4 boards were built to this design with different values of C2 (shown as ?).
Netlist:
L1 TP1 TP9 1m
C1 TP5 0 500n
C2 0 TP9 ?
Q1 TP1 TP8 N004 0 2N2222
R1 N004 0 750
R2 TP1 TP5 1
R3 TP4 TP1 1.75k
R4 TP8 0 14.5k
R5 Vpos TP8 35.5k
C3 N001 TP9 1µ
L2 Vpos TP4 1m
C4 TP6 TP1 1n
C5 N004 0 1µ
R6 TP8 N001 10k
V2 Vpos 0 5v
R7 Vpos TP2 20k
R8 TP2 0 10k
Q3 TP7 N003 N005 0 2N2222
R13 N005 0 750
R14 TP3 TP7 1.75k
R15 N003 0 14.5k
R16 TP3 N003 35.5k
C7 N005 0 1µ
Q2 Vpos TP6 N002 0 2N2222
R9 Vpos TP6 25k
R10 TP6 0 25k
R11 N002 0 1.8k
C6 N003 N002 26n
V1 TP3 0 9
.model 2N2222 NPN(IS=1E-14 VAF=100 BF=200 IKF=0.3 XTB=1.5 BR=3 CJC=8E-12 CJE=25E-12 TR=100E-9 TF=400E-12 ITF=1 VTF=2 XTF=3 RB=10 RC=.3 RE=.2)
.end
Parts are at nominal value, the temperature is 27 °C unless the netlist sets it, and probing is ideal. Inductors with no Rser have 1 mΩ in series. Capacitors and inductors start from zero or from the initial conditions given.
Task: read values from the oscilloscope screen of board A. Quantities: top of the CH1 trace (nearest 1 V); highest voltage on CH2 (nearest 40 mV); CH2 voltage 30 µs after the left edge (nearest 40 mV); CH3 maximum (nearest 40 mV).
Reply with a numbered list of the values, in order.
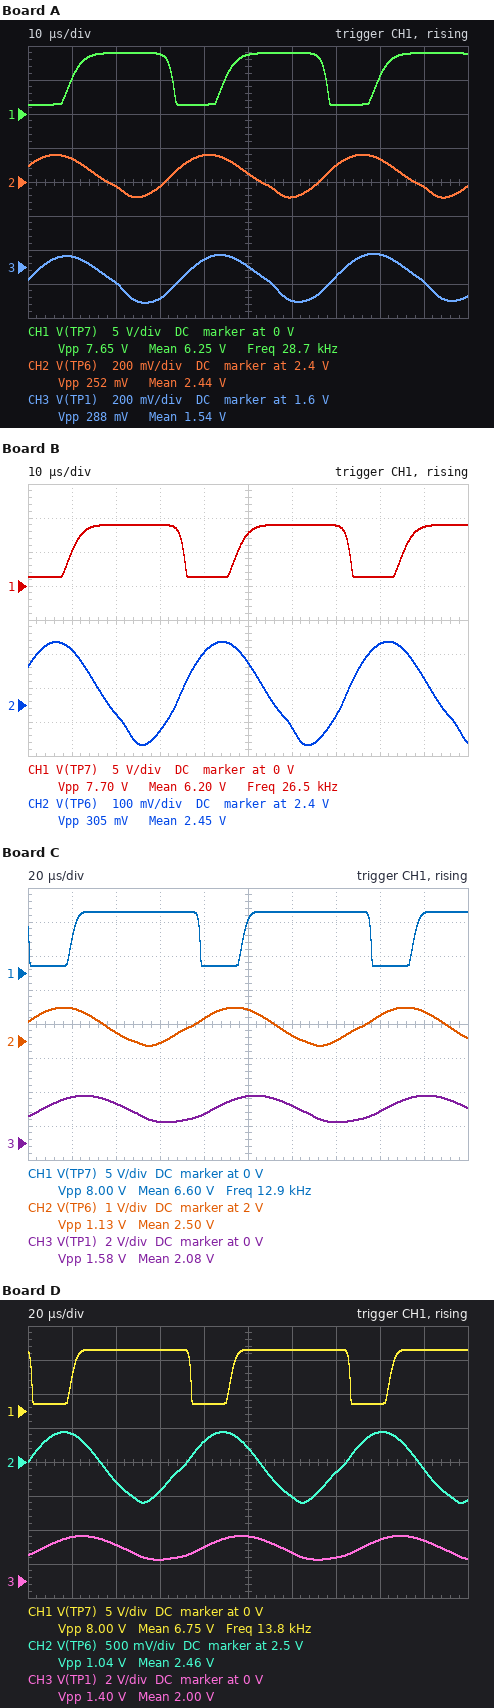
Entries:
1. 9 V
2. 2.56 V
3. 2.36 V
4. 1.68 V
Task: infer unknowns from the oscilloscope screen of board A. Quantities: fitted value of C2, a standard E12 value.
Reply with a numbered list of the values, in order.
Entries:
1. 33 nF
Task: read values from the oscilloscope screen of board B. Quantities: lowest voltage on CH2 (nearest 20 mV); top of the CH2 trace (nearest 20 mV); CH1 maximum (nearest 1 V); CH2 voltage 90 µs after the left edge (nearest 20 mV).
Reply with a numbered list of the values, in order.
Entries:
1. 2.28 V
2. 2.58 V
3. 9 V
4. 2.48 V
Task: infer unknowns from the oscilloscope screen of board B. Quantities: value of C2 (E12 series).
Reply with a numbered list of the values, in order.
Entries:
1. 39 nF
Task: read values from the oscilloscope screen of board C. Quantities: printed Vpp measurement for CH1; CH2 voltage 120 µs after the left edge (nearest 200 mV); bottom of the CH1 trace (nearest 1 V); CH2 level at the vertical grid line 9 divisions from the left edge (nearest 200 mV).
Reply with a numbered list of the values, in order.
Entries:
1. 8.00 V
2. 2.2 V
3. 1 V
4. 2.8 V
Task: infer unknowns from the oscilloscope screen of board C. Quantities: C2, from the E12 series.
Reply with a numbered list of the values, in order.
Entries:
1. 220 nF
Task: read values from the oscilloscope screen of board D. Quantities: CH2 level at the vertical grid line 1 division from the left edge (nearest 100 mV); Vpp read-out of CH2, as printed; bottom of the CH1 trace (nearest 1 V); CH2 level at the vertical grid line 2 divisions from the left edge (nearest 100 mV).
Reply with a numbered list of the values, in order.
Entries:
1. 2.9 V
2. 1.04 V
3. 1 V
4. 2.2 V
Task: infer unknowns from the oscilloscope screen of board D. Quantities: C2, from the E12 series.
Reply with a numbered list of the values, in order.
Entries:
1. 180 nF
